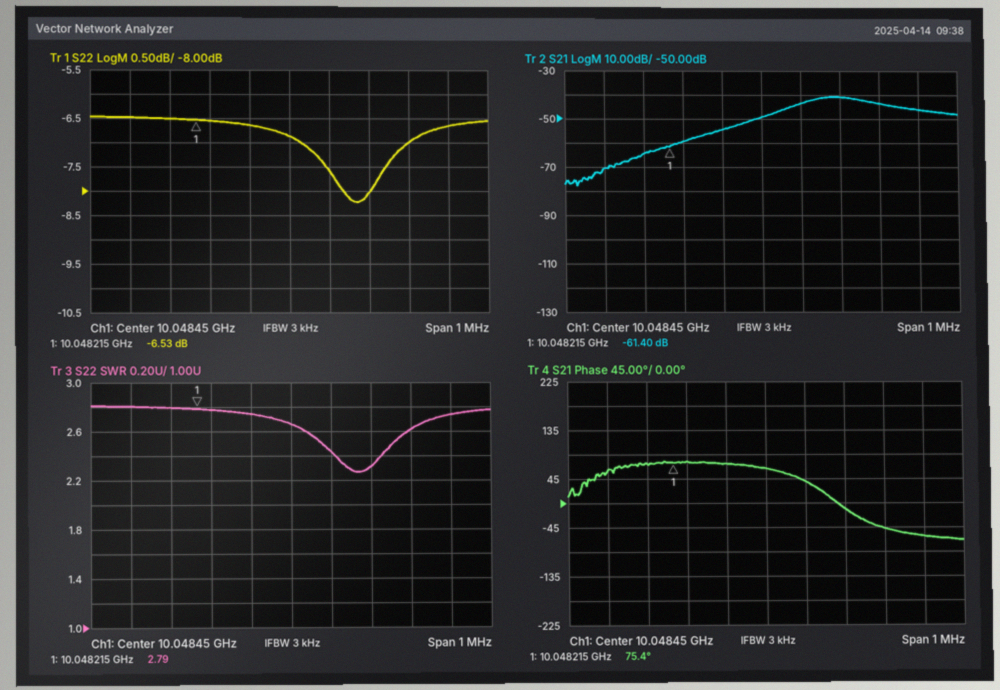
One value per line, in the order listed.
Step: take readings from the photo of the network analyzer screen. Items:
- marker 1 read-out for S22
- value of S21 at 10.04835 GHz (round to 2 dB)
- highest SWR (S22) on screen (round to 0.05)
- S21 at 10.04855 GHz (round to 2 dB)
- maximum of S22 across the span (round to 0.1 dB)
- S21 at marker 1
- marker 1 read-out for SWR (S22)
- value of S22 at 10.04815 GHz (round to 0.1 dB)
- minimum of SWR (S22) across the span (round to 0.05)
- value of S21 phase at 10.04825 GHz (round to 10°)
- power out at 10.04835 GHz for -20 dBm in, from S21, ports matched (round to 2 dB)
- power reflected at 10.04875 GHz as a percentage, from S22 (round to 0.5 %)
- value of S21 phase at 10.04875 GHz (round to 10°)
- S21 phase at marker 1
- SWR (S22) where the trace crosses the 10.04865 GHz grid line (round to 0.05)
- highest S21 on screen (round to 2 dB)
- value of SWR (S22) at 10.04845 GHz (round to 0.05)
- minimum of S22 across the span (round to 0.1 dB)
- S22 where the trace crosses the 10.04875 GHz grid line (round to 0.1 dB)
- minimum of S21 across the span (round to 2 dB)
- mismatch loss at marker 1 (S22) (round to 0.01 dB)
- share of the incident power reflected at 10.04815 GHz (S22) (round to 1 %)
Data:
-6.53 dB
-54 dB
2.80
-44 dB
-6.5 dB
-61.40 dB
2.79
-6.5 dB
2.25
80°
-74 dBm
20.0 %
-50°
75.4°
2.30
-40 dB
2.65
-8.2 dB
-7.0 dB
-78 dB
1.09 dB
22 %
